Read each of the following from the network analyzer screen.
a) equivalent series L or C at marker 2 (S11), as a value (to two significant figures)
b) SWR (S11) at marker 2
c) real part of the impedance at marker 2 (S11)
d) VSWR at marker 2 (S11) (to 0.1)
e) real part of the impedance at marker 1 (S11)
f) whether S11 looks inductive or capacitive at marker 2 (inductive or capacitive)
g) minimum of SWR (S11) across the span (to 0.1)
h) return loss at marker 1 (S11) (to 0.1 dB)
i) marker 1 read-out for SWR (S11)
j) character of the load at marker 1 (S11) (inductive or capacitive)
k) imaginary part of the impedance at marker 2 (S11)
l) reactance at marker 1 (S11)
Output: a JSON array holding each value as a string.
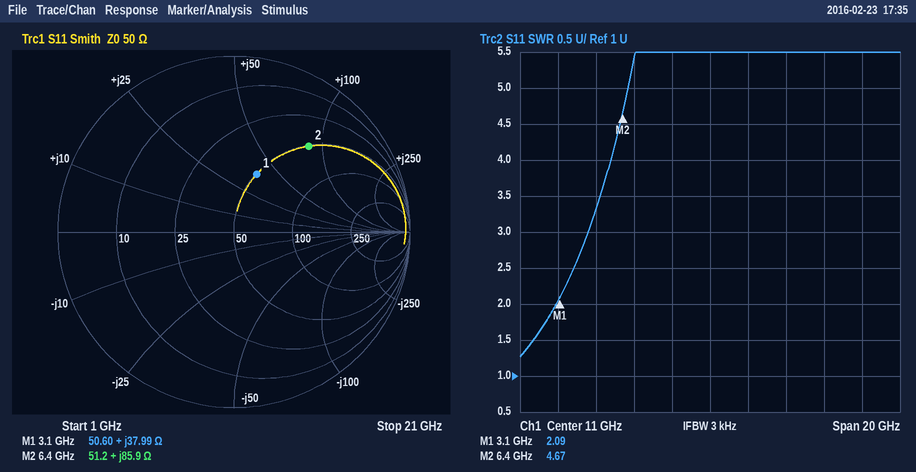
["2.1 nH", "4.67", "51.2 Ω", "4.7", "50.60 Ω", "inductive", "1.3", "9.0 dB", "2.09", "inductive", "+85.9 Ω", "+37.99 Ω"]
